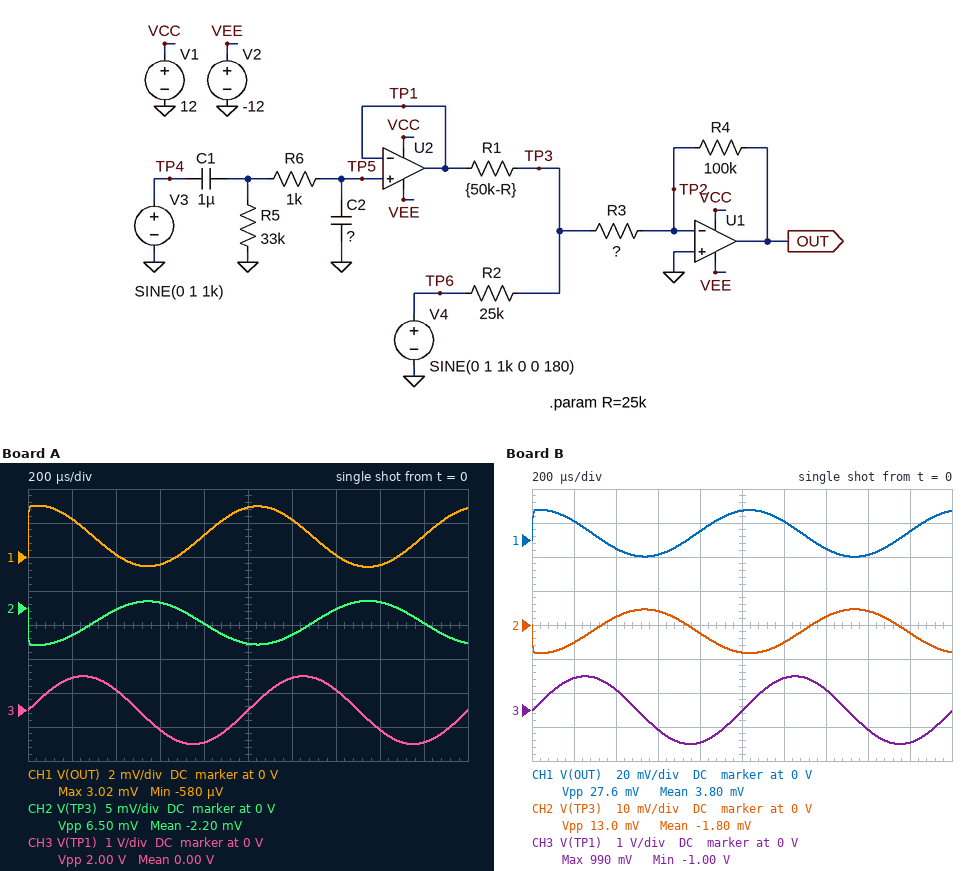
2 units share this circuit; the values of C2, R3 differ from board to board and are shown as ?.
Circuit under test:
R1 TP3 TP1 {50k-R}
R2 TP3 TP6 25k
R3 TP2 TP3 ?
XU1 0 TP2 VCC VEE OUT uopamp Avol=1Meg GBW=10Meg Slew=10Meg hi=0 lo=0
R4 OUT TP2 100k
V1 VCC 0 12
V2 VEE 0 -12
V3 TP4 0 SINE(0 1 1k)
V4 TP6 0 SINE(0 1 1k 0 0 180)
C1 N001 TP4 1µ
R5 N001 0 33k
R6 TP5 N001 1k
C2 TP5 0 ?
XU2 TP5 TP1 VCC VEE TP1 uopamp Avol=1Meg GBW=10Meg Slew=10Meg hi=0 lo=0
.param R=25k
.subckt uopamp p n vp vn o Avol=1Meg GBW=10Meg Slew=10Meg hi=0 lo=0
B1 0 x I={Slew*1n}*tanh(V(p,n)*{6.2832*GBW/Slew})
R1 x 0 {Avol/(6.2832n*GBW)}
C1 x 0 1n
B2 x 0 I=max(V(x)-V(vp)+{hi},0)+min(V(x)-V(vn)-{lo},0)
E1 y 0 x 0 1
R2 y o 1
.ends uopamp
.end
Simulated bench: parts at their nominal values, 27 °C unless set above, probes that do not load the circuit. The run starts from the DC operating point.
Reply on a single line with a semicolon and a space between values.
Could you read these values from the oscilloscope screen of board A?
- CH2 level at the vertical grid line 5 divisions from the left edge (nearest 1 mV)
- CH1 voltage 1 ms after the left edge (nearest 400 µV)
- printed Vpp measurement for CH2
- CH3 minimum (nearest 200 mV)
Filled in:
-5 mV; 2.8 mV; 6.50 mV; -1.0 V
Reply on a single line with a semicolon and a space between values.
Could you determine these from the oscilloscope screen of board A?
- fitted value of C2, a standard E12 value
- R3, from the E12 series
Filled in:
1.8 nF; 180 kΩ
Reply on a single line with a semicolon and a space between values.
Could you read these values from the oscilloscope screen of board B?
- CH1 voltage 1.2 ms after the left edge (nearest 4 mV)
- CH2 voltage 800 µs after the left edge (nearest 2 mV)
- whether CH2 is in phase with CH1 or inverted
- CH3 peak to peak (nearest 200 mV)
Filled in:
12 mV; -2 mV; inverted; 2.0 V
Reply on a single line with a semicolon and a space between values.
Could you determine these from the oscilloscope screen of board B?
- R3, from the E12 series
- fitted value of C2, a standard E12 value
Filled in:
47 kΩ; 3.3 nF
